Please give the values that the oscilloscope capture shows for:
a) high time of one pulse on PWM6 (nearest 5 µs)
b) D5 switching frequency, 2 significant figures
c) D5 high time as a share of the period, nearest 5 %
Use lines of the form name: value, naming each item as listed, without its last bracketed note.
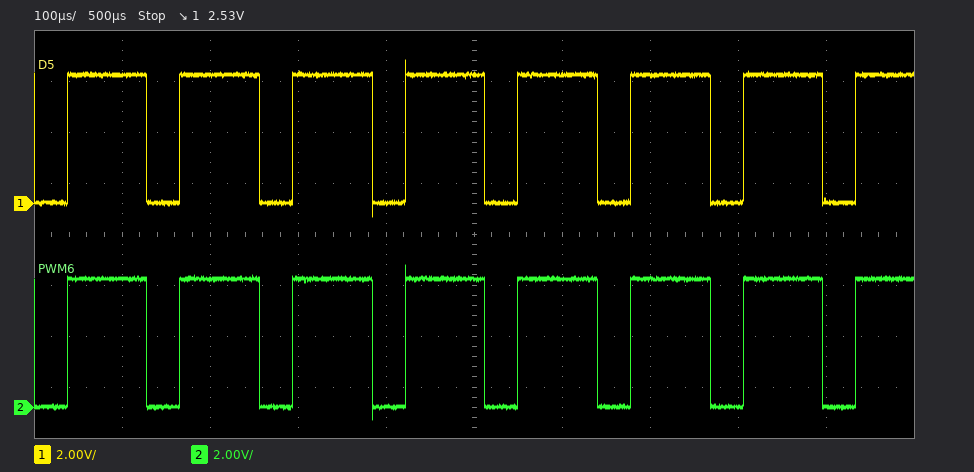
high time of one pulse on PWM6: 90 µs
D5 switching frequency, 2 significant figures: 7.8 kHz
D5 high time as a share of the period, nearest 5 %: 70 %
